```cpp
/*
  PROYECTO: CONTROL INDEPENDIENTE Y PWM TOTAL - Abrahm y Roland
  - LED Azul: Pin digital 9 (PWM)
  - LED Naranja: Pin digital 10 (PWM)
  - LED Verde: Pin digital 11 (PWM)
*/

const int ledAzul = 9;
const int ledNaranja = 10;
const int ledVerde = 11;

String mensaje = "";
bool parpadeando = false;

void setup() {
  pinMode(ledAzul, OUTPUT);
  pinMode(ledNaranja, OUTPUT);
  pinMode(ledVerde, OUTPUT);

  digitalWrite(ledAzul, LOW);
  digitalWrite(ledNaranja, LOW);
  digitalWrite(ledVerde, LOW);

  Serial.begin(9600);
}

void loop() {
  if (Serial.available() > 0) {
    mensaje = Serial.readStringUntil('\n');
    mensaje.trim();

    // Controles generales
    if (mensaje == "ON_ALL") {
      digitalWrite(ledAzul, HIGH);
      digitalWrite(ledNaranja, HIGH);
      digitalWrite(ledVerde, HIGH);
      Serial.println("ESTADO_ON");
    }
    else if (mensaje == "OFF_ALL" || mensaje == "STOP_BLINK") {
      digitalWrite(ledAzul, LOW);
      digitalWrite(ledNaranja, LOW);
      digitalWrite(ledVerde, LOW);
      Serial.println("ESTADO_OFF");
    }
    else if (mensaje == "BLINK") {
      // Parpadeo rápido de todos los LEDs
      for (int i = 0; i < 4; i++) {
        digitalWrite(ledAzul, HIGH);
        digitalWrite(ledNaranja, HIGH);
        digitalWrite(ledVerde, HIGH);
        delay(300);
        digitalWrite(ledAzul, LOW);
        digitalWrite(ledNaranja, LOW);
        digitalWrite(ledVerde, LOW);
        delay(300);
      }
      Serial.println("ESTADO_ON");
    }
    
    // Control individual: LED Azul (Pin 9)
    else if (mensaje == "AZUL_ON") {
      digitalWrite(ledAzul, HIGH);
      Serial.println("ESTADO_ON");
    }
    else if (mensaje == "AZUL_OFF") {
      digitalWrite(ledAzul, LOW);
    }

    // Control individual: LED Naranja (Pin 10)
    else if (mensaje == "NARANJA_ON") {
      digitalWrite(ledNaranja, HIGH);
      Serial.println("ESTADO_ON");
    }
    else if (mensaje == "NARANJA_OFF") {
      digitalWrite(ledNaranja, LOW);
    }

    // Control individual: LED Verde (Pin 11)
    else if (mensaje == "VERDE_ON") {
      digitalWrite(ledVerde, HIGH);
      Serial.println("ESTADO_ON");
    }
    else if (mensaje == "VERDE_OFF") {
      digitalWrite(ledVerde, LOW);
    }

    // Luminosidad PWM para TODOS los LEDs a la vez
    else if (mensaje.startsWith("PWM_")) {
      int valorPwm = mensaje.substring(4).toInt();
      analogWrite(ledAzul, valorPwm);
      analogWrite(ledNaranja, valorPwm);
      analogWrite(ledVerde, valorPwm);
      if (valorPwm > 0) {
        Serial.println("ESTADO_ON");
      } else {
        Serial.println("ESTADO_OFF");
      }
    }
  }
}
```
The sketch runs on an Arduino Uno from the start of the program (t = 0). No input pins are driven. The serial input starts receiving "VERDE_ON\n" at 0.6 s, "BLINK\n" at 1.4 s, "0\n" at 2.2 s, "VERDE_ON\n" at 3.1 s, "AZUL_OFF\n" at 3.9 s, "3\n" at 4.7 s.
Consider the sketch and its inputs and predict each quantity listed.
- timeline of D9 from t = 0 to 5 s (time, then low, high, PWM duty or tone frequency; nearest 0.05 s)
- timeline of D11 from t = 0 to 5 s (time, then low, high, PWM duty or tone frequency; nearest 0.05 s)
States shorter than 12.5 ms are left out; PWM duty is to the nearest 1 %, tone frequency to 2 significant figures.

0 s low; 1.4 s high; 1.7 s low; 2 s high; 2.3 s low; 2.6 s high; 2.9 s low; 3.2 s high; 3.5 s low
0 s low; 0.6 s high; 1.7 s low; 2 s high; 2.3 s low; 2.6 s high; 2.9 s low; 3.2 s high; 3.5 s low; 3.8 s high
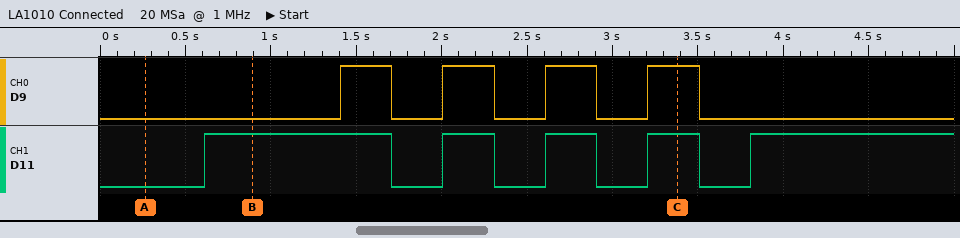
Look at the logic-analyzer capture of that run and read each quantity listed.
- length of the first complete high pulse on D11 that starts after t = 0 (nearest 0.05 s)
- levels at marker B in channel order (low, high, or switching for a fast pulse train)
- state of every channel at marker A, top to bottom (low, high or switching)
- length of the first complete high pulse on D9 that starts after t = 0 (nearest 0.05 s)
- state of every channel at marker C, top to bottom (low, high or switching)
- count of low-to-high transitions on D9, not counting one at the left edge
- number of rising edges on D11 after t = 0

1.10 s
D9 low, D11 high
D9 low, D11 low
0.30 s
D9 high, D11 high
4
5
